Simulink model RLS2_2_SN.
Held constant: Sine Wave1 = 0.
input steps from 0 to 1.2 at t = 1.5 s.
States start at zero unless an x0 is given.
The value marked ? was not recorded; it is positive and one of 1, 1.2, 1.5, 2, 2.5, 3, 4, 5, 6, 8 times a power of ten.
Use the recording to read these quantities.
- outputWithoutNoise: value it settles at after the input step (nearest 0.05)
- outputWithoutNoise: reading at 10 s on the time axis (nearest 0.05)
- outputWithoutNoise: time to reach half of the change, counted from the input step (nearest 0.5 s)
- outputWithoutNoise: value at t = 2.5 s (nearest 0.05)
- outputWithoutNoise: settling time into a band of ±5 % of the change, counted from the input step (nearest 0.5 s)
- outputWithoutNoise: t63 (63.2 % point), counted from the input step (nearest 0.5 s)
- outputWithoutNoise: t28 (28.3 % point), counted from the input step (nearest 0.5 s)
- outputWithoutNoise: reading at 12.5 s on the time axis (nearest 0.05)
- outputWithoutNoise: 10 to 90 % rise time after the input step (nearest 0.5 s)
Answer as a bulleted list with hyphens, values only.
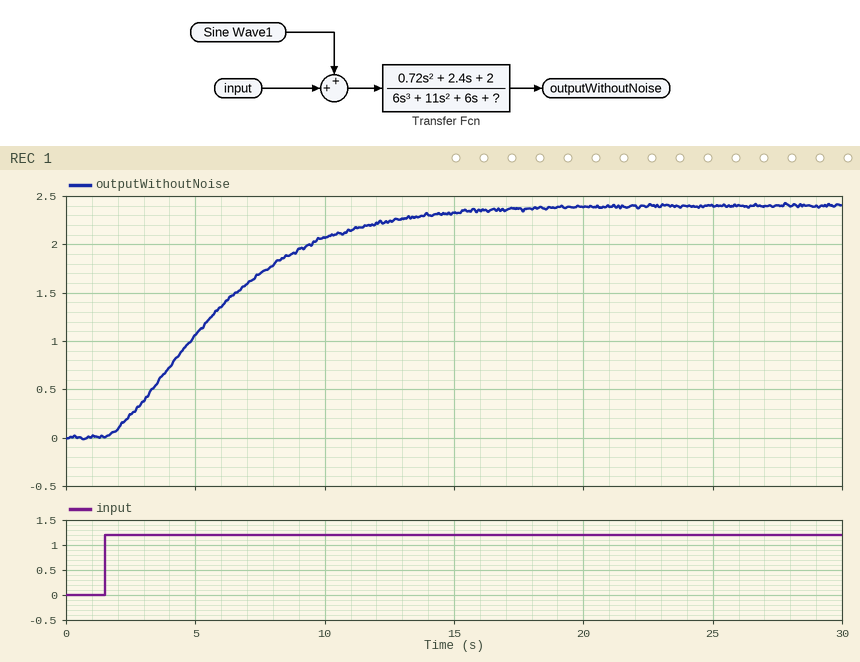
- 2.40
- 2.05
- 4.0 s
- 0.25
- 12.0 s
- 5.0 s
- 2.5 s
- 2.25
- 8.5 s
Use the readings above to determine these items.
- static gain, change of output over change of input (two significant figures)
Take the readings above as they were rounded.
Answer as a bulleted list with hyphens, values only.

- 2.0
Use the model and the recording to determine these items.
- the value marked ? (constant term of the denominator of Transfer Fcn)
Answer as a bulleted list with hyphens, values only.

- 1
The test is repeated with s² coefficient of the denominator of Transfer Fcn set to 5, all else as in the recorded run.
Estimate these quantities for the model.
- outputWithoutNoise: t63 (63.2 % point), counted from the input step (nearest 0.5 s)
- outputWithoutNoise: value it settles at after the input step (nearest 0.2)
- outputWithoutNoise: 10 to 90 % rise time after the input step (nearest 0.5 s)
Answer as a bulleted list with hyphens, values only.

- 4.0 s
- 2.4
- 10.5 s
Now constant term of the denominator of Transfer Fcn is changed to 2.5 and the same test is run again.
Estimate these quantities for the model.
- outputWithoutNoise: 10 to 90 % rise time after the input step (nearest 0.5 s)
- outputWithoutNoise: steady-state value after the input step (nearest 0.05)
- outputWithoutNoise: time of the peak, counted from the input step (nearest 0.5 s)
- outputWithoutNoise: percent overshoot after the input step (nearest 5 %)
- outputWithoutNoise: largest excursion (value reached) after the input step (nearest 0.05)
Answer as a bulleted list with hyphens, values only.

- 2.5 s
- 0.95
- 6.0 s
- 20 %
- 1.15
